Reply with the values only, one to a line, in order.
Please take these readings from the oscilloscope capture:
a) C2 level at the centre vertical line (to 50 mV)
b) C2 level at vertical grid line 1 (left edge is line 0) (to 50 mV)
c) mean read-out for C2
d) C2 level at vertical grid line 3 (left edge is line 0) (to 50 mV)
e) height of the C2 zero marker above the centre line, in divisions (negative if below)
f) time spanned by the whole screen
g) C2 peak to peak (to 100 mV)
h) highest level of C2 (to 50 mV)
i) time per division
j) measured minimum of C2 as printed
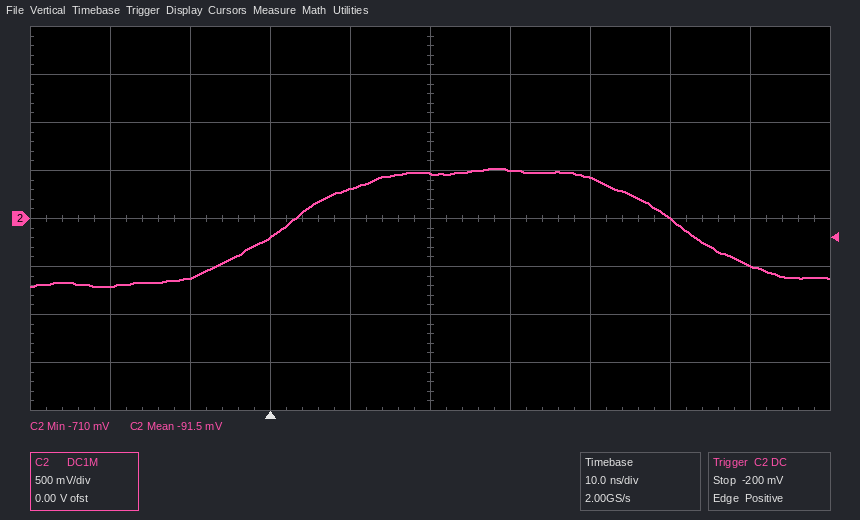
450 mV
-700 mV
-91.5 mV
-200 mV
0.0 div
100 ns
1.20 V
500 mV
10 ns
-710 mV
